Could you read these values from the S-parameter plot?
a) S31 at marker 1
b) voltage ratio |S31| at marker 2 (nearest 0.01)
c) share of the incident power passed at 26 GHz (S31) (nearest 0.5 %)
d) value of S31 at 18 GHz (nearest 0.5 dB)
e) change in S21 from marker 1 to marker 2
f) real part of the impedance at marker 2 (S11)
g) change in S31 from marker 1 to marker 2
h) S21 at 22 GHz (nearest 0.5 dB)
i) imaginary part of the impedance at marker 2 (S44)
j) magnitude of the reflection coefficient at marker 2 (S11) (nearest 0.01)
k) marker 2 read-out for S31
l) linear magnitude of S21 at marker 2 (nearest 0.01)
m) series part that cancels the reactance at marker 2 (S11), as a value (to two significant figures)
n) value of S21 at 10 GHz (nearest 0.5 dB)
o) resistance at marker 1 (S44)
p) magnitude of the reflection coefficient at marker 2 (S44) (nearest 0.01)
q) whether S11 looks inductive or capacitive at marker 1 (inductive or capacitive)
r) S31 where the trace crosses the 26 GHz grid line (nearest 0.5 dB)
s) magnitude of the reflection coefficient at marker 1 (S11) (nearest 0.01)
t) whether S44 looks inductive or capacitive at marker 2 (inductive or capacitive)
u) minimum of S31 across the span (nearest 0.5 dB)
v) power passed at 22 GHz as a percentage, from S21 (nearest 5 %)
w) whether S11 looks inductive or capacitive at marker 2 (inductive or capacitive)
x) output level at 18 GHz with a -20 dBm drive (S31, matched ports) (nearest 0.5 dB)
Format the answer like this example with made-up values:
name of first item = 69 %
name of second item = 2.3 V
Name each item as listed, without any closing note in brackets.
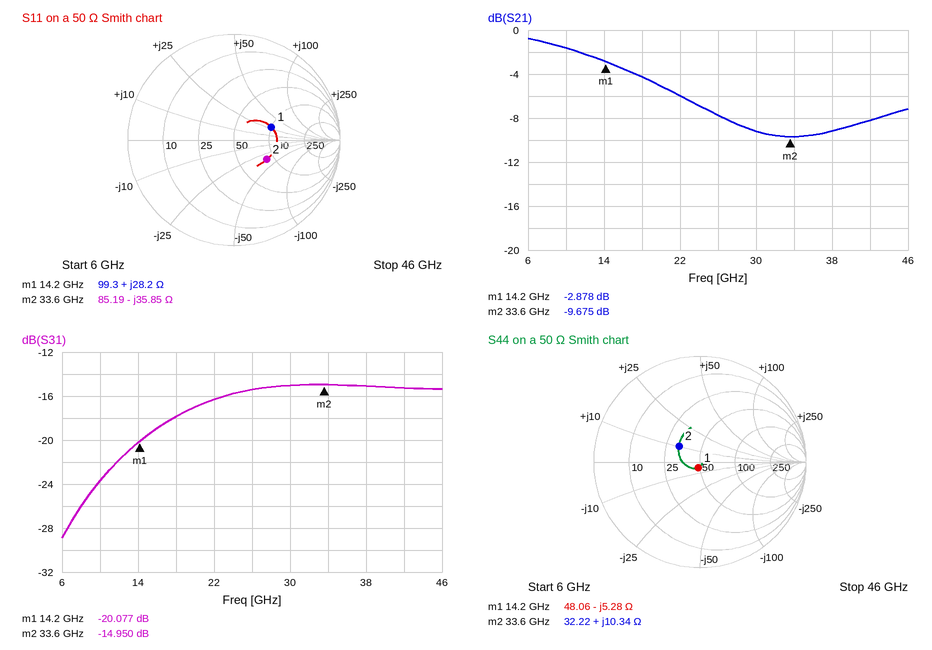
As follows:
S31 at marker 1 = -20.077 dB
voltage ratio |S31| at marker 2 = 0.18
share of the incident power passed at 26 GHz (S31) = 3.0 %
value of S31 at 18 GHz = -18.0 dB
change in S21 from marker 1 to marker 2 = -6.797 dB
real part of the impedance at marker 2 = 85.19 Ω
change in S31 from marker 1 to marker 2 = 5.127 dB
S21 at 22 GHz = -6.0 dB
imaginary part of the impedance at marker 2 = +10.34 Ω
magnitude of the reflection coefficient at marker 2 (S11) = 0.36
marker 2 read-out for S31 = -14.950 dB
linear magnitude of S21 at marker 2 = 0.33
series part that cancels the reactance at marker 2 (S11), as a value = 170 pH
value of S21 at 10 GHz = -1.5 dB
resistance at marker 1 = 48.06 Ω
magnitude of the reflection coefficient at marker 2 (S44) = 0.25
whether S11 looks inductive or capacitive at marker 1 = inductive
S31 where the trace crosses the 26 GHz grid line = -15.5 dB
magnitude of the reflection coefficient at marker 1 (S11) = 0.37
whether S44 looks inductive or capacitive at marker 2 = inductive
minimum of S31 across the span = -29.0 dB
power passed at 22 GHz as a percentage, from S21 = 25 %
whether S11 looks inductive or capacitive at marker 2 = capacitive
output level at 18 GHz with a -20 dBm drive (S31, matched ports) = -38.0 dBm
